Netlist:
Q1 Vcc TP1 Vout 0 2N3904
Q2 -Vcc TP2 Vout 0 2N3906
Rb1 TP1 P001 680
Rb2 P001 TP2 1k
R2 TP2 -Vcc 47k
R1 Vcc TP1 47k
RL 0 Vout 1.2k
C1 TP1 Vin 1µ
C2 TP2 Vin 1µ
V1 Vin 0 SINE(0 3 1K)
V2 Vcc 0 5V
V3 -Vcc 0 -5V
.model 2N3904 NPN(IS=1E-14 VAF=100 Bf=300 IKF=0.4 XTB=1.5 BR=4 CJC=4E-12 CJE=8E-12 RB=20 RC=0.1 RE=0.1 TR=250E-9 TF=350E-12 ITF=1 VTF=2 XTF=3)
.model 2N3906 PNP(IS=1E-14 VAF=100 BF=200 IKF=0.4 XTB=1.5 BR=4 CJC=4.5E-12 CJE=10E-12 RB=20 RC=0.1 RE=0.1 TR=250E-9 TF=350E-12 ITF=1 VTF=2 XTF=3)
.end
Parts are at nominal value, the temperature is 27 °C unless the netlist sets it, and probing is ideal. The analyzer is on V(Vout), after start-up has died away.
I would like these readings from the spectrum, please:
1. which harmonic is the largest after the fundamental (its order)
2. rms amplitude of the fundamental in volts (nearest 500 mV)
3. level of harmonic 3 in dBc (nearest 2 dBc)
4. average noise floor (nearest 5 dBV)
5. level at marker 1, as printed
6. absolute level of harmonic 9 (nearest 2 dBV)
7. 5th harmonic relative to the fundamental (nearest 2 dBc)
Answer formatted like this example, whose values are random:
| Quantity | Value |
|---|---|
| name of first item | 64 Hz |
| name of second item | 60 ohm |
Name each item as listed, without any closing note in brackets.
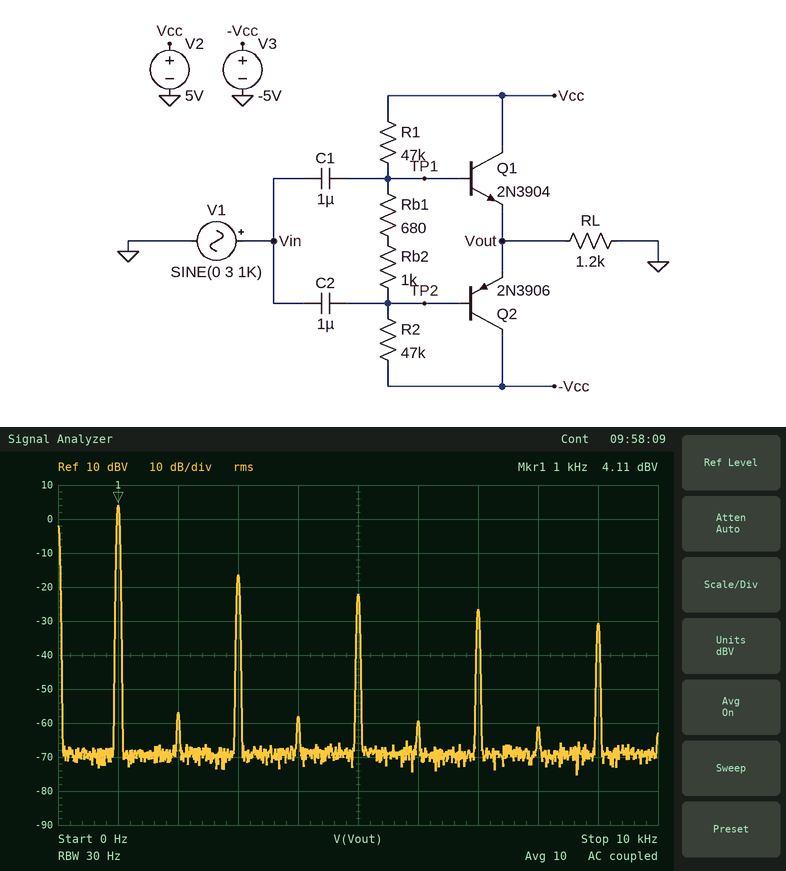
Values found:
| Quantity | Value |
|---|---|
| which harmonic is the largest after the fundamental | 3 |
| rms amplitude of the fundamental in volts | 1.5 V |
| level of harmonic 3 in dBc | -20 dBc |
| average noise floor | -70 dBV |
| level at marker 1, as printed | 4.11 dBV |
| absolute level of harmonic 9 | -30 dBV |
| 5th harmonic relative to the fundamental | -26 dBc |
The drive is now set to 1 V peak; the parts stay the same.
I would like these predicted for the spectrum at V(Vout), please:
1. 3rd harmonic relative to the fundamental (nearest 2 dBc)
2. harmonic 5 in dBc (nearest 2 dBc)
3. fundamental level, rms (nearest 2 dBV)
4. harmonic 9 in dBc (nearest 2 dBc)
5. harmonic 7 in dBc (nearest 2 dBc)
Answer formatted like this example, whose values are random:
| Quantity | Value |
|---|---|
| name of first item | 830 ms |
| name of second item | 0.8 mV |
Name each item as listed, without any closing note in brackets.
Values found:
| Quantity | Value |
|---|---|
| 3rd harmonic relative to the fundamental | -10 dBc |
| harmonic 5 in dBc | -24 dBc |
| fundamental level, rms | -12 dBV |
| harmonic 9 in dBc | -32 dBc |
| harmonic 7 in dBc | -36 dBc |
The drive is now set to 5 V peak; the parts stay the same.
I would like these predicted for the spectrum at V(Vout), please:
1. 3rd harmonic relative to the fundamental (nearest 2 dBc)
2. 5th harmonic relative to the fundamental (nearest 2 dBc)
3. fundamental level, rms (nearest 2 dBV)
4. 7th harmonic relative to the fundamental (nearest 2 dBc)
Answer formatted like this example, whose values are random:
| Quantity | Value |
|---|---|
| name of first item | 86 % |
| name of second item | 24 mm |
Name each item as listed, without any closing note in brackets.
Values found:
| Quantity | Value |
|---|---|
| 3rd harmonic relative to the fundamental | -26 dBc |
| 5th harmonic relative to the fundamental | -30 dBc |
| fundamental level, rms | 10 dBV |
| 7th harmonic relative to the fundamental | -34 dBc |
